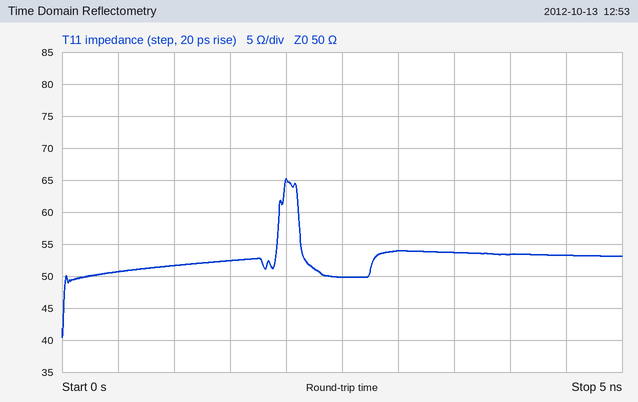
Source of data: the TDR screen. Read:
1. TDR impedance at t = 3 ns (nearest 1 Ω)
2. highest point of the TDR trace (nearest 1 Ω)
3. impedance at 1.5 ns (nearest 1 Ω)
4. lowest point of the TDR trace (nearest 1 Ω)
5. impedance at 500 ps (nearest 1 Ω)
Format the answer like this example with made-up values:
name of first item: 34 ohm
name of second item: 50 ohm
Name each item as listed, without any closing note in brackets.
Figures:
TDR impedance at t = 3 ns: 54 Ω
highest point of the TDR trace: 65 Ω
impedance at 1.5 ns: 52 Ω
lowest point of the TDR trace: 40 Ω
impedance at 500 ps: 51 Ω
